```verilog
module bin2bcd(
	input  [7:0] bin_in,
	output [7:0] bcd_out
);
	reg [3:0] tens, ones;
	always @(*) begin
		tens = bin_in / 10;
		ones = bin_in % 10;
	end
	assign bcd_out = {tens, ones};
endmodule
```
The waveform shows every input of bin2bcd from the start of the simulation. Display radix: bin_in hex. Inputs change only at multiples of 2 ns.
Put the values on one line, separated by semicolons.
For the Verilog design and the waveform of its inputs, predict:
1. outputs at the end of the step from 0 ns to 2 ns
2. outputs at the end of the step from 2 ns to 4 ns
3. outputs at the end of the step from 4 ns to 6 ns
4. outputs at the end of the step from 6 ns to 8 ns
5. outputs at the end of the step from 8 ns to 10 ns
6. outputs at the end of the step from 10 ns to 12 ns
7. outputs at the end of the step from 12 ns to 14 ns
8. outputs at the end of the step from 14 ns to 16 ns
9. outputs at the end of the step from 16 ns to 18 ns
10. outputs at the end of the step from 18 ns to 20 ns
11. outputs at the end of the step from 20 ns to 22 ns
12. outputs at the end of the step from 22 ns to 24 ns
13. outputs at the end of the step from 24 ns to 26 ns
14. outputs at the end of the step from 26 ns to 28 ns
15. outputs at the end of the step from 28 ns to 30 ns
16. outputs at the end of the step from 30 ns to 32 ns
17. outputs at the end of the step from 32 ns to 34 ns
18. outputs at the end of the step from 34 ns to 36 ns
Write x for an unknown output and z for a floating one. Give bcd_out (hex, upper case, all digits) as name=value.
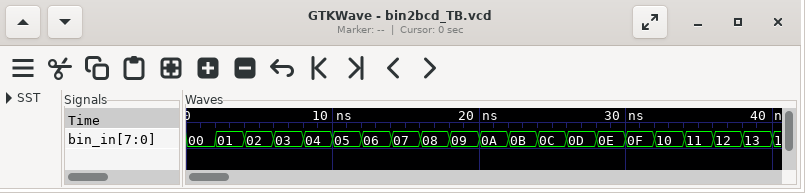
bcd_out=00; bcd_out=01; bcd_out=02; bcd_out=03; bcd_out=04; bcd_out=05; bcd_out=06; bcd_out=07; bcd_out=08; bcd_out=09; bcd_out=10; bcd_out=11; bcd_out=12; bcd_out=13; bcd_out=14; bcd_out=15; bcd_out=16; bcd_out=17
